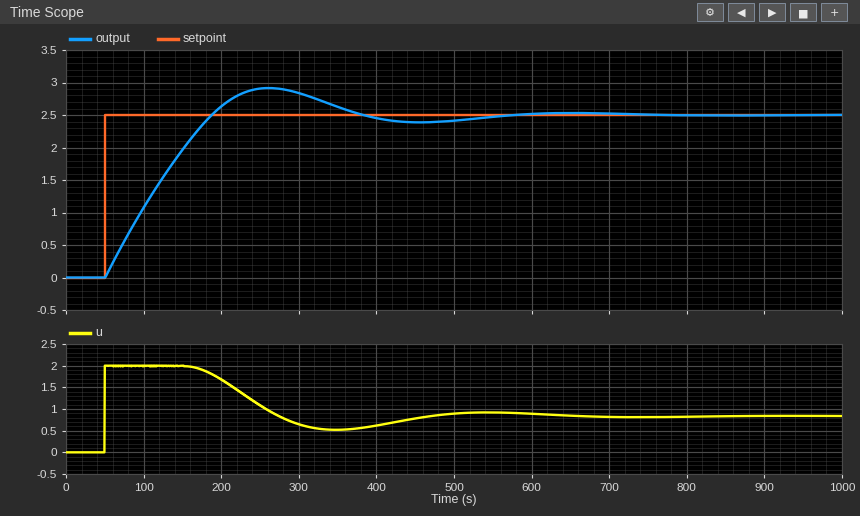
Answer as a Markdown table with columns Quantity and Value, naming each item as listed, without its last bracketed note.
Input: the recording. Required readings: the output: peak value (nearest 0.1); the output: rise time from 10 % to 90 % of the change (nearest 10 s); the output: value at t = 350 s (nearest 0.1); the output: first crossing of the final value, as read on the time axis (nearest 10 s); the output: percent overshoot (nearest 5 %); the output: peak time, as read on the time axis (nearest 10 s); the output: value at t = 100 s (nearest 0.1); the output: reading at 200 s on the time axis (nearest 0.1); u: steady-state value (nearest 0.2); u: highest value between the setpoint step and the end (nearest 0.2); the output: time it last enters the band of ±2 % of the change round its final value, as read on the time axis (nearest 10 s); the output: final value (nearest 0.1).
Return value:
| Quantity | Value |
|---|---|
| the output: peak value | 2.9 |
| the output: rise time from 10 % to 90 % of the change | 110 s |
| the output: value at t = 350 s | 2.6 |
| the output: first crossing of the final value, as read on the time axis | 190 s |
| the output: percent overshoot | 15 % |
| the output: peak time, as read on the time axis | 260 s |
| the output: value at t = 100 s | 1.1 |
| the output: reading at 200 s on the time axis | 2.6 |
| u: steady-state value | 0.8 |
| u: highest value between the setpoint step and the end | 2.0 |
| the output: time it last enters the band of ±2 % of the change round its final value, as read on the time axis | 530 s |
| the output: final value | 2.5 |
